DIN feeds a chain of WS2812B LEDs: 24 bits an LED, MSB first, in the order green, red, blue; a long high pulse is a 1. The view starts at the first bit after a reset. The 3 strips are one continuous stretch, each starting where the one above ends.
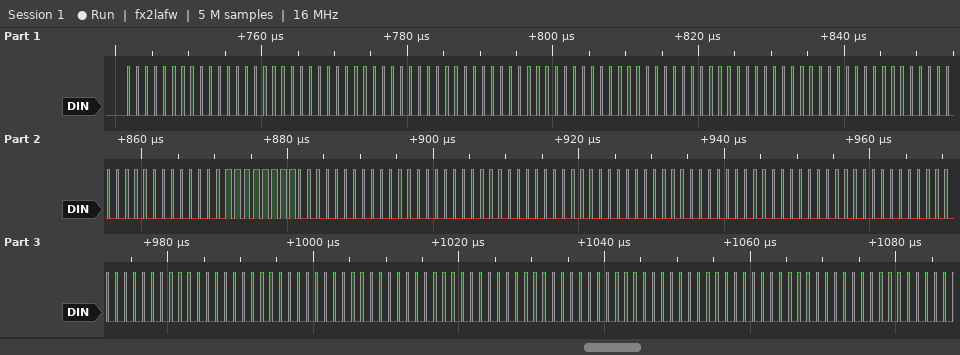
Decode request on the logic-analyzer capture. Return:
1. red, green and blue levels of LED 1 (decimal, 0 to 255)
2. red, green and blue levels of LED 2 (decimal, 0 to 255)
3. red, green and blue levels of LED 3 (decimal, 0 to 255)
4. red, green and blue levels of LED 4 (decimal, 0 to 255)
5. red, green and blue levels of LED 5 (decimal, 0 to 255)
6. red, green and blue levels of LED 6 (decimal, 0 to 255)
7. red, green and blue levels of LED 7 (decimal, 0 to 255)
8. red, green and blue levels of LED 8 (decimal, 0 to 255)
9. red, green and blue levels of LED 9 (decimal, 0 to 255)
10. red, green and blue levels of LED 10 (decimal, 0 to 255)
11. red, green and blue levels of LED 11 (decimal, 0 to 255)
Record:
0, 0, 0
0, 0, 0
0, 0, 0
0, 0, 0
255, 0, 0
0, 0, 0
0, 0, 0
0, 0, 0
0, 0, 0
0, 0, 0
0, 0, 0
